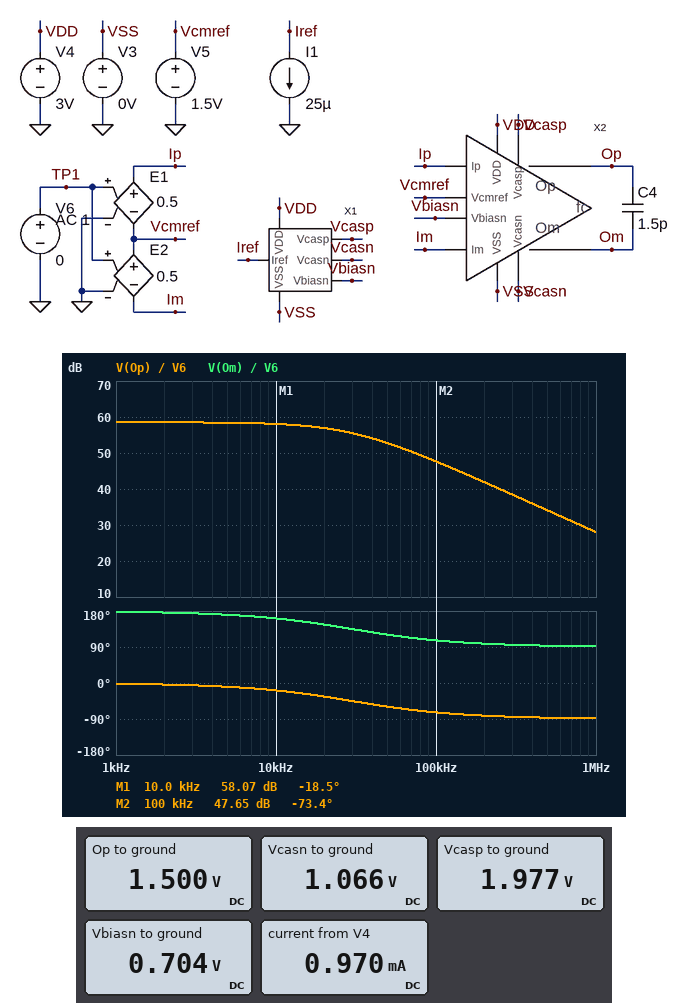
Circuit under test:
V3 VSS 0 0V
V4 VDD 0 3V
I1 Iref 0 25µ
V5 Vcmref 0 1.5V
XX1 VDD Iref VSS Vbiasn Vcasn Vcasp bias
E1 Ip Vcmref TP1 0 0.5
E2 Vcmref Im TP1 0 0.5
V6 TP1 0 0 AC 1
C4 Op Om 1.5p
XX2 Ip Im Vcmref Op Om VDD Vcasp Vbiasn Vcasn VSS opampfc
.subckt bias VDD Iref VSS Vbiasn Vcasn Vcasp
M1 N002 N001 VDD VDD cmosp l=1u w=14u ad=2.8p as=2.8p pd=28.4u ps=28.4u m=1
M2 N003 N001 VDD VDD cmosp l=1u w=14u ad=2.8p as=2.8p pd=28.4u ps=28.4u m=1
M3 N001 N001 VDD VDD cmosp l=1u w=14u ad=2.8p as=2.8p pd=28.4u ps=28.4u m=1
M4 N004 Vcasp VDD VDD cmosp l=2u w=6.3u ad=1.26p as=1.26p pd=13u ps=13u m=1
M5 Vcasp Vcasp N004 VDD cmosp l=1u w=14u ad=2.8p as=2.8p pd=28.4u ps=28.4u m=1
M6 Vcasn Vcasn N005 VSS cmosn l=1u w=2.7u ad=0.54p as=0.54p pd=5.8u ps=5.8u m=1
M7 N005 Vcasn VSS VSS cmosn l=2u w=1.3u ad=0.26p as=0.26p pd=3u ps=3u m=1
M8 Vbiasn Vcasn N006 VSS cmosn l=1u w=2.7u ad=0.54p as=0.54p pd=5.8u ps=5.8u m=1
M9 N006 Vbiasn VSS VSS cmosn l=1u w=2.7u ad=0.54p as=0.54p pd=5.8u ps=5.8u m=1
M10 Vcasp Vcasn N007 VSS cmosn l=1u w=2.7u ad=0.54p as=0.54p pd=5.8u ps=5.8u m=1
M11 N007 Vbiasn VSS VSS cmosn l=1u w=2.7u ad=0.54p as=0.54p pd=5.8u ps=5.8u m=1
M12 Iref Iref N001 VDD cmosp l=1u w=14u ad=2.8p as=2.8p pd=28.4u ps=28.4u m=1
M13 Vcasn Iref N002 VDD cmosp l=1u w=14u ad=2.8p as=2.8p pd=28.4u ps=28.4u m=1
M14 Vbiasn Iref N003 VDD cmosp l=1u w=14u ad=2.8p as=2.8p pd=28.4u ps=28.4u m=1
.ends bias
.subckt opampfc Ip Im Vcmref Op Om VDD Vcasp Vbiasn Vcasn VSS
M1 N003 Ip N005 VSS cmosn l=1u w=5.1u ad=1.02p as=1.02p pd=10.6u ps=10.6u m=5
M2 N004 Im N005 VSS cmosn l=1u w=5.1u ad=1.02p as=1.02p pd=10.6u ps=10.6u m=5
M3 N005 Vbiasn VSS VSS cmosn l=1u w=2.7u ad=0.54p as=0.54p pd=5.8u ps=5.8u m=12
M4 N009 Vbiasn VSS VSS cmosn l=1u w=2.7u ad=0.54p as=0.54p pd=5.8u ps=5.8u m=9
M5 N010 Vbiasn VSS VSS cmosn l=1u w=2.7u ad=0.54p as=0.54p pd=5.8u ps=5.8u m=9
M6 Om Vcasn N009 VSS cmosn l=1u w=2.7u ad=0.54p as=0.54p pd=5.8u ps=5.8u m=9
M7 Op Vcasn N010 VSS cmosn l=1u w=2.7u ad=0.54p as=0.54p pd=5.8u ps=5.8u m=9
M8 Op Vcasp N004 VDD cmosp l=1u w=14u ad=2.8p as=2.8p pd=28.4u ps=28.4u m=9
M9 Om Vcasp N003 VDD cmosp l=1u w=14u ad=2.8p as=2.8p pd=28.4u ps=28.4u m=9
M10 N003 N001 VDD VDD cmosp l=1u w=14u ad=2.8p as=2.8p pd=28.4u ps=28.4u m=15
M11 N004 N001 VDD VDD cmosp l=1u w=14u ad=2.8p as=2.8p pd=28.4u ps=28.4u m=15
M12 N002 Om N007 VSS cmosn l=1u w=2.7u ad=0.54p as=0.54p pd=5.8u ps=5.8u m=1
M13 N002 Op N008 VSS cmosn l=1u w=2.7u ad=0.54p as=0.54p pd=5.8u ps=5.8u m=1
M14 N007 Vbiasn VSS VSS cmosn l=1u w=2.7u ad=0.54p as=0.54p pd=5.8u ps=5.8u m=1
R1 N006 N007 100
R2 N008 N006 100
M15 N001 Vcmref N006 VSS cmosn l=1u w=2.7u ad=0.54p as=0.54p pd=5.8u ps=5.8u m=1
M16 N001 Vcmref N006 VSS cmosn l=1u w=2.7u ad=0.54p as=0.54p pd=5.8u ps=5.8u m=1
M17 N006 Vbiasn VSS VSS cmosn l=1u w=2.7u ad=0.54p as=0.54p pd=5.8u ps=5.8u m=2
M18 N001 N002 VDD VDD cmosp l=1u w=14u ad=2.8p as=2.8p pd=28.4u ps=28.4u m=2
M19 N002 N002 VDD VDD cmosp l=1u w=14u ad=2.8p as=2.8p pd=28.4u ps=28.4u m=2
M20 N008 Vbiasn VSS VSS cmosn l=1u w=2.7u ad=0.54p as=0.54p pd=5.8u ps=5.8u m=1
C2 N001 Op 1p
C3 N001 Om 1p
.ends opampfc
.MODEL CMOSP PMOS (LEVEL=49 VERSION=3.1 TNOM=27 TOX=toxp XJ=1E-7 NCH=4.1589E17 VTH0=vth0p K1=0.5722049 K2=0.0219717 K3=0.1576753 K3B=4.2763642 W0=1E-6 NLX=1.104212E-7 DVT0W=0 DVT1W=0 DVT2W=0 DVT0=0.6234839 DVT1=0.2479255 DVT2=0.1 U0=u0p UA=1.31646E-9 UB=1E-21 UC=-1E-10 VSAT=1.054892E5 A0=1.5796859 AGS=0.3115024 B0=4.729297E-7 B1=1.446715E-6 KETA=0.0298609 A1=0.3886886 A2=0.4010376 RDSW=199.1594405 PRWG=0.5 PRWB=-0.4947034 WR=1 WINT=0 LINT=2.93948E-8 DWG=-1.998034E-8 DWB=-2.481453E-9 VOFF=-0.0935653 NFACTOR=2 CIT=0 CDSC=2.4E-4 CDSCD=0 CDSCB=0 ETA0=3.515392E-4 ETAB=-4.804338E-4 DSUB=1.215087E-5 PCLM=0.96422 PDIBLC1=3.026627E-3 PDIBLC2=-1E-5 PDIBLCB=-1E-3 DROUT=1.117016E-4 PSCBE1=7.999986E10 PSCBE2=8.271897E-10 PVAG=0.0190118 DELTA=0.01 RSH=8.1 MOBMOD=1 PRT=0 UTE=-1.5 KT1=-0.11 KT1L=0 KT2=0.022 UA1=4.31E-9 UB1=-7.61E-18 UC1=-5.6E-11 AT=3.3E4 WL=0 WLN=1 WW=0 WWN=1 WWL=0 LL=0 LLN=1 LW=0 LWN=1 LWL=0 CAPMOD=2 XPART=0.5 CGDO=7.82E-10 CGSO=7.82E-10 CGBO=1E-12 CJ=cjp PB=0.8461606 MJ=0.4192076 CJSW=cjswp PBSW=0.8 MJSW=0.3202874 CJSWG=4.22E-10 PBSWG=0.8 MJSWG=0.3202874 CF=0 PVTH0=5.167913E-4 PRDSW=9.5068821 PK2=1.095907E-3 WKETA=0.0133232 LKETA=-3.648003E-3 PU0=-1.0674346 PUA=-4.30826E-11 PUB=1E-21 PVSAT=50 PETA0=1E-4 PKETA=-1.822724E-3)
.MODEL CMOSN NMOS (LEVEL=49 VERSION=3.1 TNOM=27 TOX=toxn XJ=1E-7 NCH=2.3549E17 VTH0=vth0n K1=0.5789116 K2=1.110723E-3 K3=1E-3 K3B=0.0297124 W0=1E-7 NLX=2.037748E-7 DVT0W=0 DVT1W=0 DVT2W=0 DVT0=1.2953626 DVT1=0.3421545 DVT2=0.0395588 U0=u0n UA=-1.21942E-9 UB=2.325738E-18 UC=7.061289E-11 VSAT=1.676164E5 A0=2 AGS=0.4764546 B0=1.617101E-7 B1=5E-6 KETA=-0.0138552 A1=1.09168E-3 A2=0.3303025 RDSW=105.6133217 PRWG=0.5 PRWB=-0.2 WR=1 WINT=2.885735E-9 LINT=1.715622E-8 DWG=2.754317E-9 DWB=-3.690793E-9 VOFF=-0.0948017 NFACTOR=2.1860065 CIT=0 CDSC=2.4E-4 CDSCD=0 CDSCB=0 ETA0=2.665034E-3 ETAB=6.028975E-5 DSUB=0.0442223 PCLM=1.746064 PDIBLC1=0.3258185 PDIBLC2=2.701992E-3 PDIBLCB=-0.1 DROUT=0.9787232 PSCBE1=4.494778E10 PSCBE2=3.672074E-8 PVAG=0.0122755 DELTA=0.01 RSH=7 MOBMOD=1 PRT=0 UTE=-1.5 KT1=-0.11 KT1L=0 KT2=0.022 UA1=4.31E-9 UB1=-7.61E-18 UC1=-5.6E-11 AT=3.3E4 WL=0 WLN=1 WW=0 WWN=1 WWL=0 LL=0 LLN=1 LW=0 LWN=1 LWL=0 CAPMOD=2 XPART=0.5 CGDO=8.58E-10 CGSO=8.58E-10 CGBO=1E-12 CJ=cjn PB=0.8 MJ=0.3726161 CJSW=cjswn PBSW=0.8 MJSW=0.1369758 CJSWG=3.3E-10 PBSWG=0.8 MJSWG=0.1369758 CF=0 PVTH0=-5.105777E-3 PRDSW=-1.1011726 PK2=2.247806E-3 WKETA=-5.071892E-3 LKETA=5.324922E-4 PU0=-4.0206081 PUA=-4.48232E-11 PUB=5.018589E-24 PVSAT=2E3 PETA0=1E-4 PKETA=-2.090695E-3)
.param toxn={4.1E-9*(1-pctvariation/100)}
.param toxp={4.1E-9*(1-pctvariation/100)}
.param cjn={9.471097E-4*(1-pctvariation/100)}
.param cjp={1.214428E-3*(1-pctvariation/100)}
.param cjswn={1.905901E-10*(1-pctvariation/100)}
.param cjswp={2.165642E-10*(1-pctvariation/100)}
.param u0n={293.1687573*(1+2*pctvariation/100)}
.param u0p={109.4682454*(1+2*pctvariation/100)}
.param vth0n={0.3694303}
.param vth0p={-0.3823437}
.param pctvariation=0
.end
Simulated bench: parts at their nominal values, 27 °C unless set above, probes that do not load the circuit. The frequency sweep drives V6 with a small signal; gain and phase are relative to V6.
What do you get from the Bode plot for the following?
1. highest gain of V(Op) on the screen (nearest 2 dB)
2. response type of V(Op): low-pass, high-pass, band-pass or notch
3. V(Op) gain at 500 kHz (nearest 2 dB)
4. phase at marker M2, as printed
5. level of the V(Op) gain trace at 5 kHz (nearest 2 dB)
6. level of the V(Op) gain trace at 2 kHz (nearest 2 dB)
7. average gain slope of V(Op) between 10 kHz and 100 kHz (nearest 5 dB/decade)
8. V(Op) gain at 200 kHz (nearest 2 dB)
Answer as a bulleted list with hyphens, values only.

- 58 dB
- low-pass
- 34 dB
- -73.4 deg
- 58 dB
- 58 dB
- -10 dB/decade
- 42 dB
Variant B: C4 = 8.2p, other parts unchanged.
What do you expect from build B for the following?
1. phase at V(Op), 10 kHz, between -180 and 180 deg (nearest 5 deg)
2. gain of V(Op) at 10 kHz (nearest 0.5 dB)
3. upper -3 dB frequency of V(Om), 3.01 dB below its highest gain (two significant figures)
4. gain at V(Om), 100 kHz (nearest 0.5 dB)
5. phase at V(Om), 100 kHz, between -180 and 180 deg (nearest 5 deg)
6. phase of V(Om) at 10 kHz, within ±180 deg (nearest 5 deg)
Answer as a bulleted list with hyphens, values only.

- -55 deg
- 54.0 dB
- 7.2 kHz
- 35.5 dB
- 95 deg
- 125 deg
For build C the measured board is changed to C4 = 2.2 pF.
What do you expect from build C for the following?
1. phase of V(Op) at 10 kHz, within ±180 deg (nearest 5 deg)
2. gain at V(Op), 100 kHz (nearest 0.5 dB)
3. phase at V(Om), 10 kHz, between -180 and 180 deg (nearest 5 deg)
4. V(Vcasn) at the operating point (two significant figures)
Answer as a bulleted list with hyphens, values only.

- -25 deg
- 45.5 dB
- 155 deg
- 1.1 V
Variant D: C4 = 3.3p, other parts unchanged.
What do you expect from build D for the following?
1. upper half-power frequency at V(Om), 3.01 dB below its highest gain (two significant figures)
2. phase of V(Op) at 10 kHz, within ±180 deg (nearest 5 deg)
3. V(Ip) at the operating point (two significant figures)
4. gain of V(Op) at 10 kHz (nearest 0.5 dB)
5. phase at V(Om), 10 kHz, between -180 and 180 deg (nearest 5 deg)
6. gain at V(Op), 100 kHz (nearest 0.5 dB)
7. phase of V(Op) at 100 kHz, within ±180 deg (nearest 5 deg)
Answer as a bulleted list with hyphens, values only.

- 16 kHz
- -30 deg
- 1.5 V
- 57.0 dB
- 150 deg
- 42.5 dB
- -80 deg
